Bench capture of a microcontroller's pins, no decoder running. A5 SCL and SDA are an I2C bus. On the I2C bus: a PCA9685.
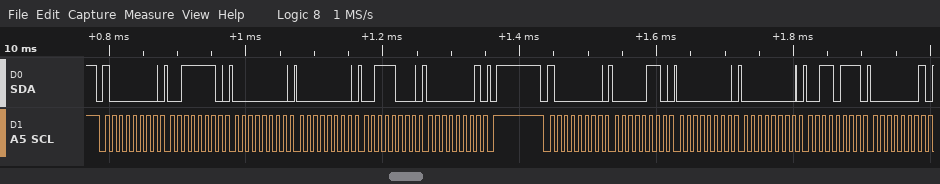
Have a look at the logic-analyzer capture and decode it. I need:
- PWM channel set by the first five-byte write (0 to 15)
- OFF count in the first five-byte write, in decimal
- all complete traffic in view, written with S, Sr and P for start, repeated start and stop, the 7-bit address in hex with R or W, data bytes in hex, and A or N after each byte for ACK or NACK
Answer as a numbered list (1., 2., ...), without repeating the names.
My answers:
1. 14
2. 312
3. S 40W A 3E A 00 A 00 A 38 A 01 A P S 40W A 06 A 00 A 00 A 37 A 01 A
